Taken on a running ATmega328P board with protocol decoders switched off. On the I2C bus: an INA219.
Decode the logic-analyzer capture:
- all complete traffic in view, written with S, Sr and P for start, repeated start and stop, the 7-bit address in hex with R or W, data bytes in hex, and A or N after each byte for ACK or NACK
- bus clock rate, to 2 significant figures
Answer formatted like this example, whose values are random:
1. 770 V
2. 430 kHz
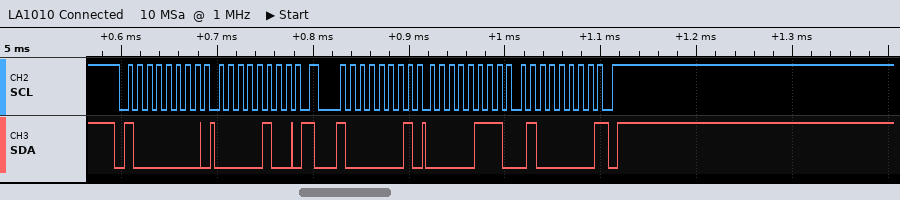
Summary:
1. S 40W A 04 A Sr 40R A 07 A 40 N P
2. 100 kHz
